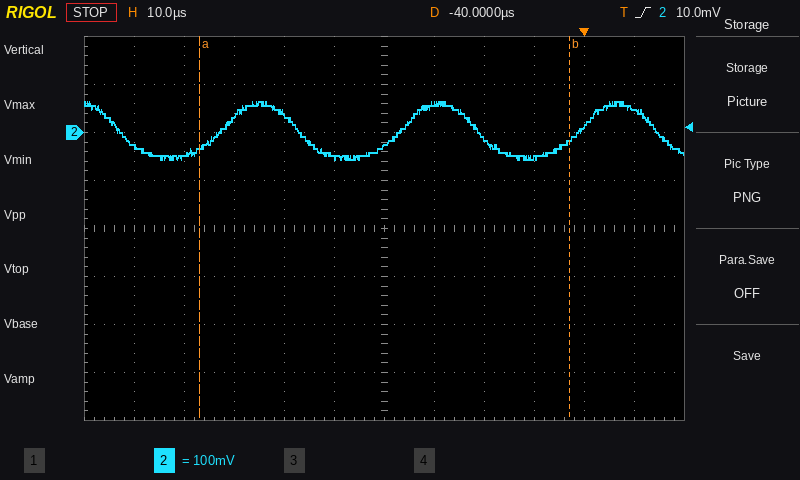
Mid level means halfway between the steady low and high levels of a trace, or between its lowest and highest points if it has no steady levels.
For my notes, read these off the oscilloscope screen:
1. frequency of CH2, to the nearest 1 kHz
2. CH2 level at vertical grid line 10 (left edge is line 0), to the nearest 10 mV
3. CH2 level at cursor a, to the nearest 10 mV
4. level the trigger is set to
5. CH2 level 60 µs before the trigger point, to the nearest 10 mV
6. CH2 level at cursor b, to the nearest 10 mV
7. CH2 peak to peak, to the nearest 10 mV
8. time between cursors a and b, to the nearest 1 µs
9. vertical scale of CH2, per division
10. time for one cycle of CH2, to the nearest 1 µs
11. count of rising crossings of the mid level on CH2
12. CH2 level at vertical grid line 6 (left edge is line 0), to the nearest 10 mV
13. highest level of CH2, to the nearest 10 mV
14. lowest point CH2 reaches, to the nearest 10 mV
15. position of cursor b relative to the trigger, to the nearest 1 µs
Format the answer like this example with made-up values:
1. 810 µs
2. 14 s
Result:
1. 28 kHz
2. 10 mV
3. -30 mV
4. 10.0 mV
5. 40 mV
6. -20 mV
7. 120 mV
8. 74 µs
9. 100 mV
10. 36 µs
11. 3
12. -30 mV
13. 60 mV
14. -60 mV
15. -3 µs
